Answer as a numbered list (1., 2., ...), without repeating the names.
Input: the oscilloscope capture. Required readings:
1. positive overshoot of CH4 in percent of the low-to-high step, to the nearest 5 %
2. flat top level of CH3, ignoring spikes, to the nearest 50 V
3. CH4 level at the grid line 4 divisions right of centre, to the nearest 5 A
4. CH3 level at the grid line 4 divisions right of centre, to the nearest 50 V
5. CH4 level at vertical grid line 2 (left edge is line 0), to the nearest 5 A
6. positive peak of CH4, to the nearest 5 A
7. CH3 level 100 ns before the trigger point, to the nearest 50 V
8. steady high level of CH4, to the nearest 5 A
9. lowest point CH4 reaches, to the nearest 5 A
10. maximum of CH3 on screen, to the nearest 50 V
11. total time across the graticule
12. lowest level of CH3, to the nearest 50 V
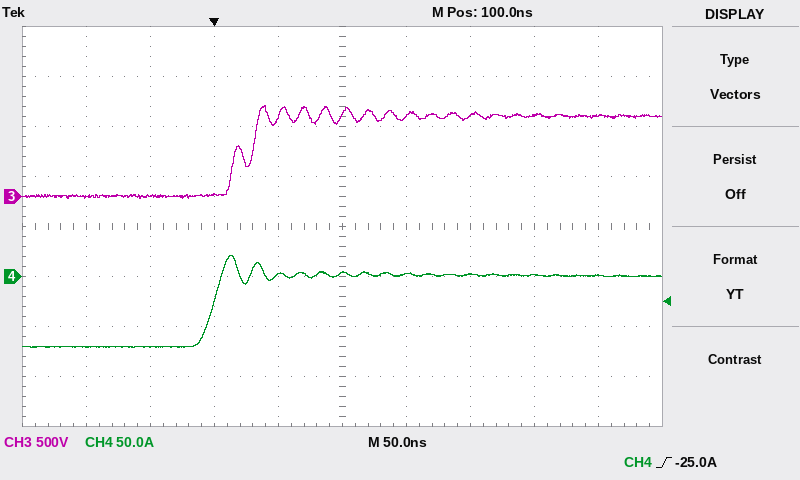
1. 30 %
2. 800 V
3. 0 A
4. 800 V
5. -70 A
6. 20 A
7. 0 V
8. 0 A
9. -70 A
10. 900 V
11. 500 ns
12. 0 V
